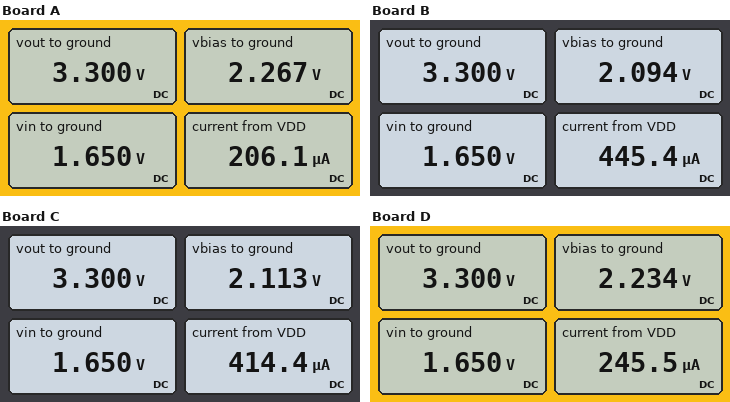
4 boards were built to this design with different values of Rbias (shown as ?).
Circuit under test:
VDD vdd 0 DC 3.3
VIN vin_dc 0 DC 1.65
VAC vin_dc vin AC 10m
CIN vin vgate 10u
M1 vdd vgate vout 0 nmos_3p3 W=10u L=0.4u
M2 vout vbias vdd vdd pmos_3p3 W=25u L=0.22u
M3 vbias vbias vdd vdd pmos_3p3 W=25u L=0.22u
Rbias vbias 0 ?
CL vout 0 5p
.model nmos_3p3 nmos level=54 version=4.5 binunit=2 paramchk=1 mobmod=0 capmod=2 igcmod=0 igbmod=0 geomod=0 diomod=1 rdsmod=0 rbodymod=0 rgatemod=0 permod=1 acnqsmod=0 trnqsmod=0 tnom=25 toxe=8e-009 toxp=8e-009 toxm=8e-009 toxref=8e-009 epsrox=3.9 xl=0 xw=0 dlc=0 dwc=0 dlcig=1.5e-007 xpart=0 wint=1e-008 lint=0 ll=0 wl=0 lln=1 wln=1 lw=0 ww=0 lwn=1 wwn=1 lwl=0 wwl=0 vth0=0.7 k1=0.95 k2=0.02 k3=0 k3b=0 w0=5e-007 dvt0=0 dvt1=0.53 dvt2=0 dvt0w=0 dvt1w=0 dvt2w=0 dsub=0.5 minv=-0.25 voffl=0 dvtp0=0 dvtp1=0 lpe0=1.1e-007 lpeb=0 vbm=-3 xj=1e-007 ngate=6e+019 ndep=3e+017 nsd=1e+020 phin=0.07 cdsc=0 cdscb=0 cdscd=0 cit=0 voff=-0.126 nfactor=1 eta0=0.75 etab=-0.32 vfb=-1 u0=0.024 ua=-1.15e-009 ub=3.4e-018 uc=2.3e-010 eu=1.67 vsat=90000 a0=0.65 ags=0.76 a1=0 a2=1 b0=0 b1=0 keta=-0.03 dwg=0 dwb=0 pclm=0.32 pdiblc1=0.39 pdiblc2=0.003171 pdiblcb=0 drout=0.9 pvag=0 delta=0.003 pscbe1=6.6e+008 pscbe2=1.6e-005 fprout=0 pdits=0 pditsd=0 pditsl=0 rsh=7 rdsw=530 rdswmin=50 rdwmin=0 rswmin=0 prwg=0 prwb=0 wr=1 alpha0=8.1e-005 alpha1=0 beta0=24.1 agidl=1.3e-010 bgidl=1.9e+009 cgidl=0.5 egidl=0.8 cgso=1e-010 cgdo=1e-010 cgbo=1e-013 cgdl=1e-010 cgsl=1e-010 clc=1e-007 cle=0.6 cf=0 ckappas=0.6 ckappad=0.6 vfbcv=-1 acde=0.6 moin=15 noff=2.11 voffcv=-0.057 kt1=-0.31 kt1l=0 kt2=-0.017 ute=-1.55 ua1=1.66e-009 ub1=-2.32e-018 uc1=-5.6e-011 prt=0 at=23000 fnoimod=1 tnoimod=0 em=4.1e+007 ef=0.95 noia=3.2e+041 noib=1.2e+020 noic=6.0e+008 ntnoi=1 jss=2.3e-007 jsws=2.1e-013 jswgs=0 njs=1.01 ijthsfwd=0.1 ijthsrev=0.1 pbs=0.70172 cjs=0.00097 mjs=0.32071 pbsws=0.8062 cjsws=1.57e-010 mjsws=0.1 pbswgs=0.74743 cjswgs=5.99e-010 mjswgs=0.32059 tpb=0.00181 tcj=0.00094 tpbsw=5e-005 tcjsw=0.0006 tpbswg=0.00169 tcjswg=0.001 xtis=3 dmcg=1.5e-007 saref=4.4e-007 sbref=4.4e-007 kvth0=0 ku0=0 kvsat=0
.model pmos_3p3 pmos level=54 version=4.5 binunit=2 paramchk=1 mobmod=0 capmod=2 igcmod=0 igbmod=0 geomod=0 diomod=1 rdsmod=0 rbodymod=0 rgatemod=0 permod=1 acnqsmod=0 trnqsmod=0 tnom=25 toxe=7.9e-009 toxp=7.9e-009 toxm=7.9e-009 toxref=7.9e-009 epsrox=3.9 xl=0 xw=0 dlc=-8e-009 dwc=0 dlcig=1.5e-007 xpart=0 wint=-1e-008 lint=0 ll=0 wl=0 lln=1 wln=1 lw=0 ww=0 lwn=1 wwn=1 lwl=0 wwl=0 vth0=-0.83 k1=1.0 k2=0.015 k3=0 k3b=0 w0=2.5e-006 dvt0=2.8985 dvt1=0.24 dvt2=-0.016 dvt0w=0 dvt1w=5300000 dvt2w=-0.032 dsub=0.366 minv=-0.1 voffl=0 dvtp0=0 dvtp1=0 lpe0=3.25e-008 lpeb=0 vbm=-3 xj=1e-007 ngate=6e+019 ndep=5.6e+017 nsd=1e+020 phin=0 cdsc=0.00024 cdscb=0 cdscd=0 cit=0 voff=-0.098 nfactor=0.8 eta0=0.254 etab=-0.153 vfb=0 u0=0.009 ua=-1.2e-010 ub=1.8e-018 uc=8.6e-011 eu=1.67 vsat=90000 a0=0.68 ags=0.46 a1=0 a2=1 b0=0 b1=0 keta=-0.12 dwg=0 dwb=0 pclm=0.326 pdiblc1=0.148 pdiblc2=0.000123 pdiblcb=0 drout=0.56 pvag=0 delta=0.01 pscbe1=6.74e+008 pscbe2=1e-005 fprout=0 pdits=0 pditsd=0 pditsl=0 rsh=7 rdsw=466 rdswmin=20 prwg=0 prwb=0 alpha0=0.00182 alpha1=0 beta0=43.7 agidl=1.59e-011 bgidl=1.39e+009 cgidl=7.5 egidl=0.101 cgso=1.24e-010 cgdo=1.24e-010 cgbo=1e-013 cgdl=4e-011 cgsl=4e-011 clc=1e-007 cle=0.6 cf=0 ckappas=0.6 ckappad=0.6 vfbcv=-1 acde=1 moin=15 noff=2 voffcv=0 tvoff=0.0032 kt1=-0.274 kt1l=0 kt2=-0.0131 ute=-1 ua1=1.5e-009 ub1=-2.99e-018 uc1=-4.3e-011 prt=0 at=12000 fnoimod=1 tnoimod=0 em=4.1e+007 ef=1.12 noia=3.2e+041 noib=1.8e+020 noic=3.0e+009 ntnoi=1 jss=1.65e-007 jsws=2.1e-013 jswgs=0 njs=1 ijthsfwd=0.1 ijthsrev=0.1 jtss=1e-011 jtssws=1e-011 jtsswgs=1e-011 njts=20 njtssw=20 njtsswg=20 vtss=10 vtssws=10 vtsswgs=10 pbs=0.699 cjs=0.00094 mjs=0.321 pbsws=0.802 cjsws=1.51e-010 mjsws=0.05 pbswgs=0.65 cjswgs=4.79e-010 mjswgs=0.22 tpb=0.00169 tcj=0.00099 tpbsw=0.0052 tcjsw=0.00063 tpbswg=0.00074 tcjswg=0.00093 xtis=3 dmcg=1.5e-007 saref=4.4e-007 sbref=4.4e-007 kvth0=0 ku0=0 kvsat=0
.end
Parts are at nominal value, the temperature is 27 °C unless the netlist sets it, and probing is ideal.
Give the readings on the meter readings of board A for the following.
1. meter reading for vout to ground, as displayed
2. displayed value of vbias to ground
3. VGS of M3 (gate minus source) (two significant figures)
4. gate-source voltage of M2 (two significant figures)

3.300 V
2.267 V
-1.0 V
-1.0 V
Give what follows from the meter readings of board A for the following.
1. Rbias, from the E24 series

11 kΩ
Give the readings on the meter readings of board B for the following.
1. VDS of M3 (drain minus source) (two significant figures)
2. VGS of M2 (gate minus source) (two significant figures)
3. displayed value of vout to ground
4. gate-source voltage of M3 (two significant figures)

-1.2 V
-1.2 V
3.300 V
-1.2 V
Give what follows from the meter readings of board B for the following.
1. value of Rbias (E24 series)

4.7 kΩ
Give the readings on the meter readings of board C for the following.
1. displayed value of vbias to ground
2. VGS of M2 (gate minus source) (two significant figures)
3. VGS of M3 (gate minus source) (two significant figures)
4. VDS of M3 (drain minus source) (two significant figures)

2.113 V
-1.2 V
-1.2 V
-1.2 V
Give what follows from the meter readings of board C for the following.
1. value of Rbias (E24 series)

5.1 kΩ
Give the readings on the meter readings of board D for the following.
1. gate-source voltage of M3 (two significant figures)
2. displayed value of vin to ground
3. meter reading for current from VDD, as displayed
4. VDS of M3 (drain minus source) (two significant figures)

-1.1 V
1.650 V
245.5 µA
-1.1 V
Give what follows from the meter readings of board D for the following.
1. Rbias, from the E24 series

9.1 kΩ
